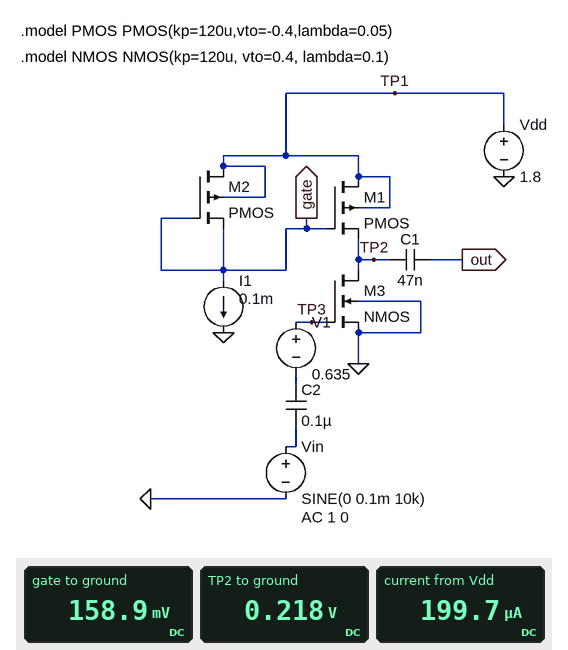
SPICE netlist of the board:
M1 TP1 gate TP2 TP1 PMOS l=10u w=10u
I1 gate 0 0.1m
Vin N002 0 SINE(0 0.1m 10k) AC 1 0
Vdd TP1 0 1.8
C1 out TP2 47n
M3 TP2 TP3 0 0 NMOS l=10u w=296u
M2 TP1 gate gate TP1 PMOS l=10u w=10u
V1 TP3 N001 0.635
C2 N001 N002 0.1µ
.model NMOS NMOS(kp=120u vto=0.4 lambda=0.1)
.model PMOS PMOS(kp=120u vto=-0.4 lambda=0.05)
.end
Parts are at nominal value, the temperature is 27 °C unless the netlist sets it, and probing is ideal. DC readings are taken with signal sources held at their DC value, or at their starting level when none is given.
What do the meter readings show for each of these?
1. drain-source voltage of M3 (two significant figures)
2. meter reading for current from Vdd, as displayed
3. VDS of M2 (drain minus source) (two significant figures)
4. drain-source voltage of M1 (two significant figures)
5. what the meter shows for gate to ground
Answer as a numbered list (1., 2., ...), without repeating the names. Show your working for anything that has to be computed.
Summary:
1. 218 mV = 220 mV
2. 199.7 µA
3. 1.8 V - 158.9 mV = 1.6 V
4. 1.8 V - 218 mV = 1.6 V
5. 158.9 mV
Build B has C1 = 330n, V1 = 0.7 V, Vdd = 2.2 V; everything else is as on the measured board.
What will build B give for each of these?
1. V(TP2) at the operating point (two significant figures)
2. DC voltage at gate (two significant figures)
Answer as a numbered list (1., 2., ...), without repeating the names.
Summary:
1. 120 mV
2. 560 mV
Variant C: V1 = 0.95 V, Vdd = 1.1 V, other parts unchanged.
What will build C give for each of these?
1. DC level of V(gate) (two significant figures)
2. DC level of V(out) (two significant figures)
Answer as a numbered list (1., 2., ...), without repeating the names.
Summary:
1. -540 mV
2. 51 mV
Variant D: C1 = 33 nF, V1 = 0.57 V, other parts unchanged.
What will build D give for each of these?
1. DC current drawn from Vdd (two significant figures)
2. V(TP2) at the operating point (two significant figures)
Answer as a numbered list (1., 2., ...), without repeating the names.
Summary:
1. 160 µA
2. 1.3 V
